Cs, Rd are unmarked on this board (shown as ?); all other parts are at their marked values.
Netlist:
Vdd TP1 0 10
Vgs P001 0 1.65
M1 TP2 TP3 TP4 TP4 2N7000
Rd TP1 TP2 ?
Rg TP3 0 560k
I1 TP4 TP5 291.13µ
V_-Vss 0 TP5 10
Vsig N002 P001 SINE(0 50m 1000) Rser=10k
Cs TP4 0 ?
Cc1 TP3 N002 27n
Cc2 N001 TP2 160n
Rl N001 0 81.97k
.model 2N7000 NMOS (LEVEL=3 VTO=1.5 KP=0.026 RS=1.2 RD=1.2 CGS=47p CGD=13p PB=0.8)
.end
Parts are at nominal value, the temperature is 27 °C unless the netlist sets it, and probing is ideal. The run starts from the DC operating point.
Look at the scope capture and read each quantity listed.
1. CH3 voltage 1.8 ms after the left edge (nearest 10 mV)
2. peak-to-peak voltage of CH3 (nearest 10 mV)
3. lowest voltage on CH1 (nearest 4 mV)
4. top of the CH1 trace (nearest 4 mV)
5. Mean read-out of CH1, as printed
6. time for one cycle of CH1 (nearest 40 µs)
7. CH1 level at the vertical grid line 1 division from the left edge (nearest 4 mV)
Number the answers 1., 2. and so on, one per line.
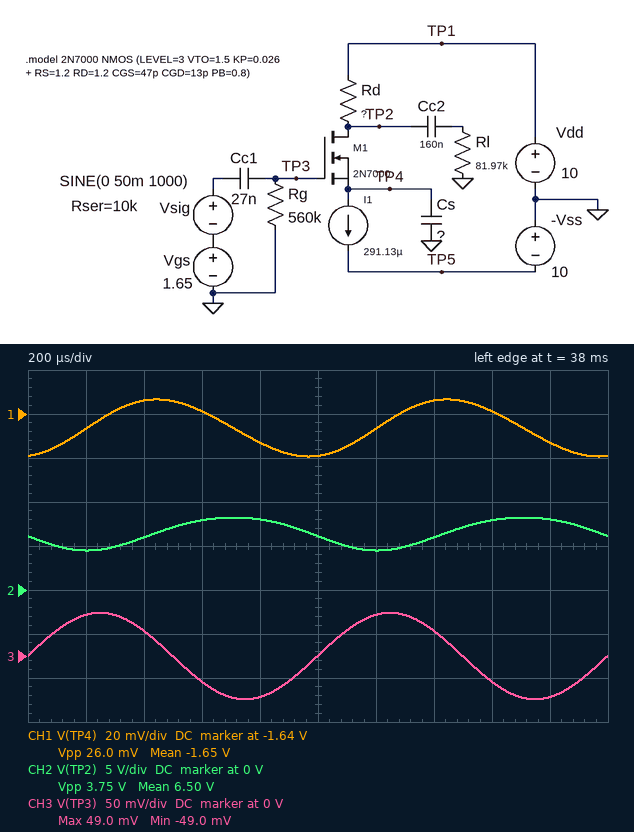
1. -50 mV
2. 100 mV
3. -1.660 V
4. -1.632 V
5. -1.65 V
6. 1.00 ms
7. -1.648 V
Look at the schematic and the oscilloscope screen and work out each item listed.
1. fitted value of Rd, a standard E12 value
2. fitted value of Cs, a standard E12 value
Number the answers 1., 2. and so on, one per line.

1. 12 kΩ
2. 2.2 µF
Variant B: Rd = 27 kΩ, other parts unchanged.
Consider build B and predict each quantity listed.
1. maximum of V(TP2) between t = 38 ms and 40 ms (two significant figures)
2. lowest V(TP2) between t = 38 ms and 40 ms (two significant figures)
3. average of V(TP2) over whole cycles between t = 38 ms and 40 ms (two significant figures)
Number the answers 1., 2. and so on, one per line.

1. 5.5 V
2. -1.5 V
3. 2.1 V
